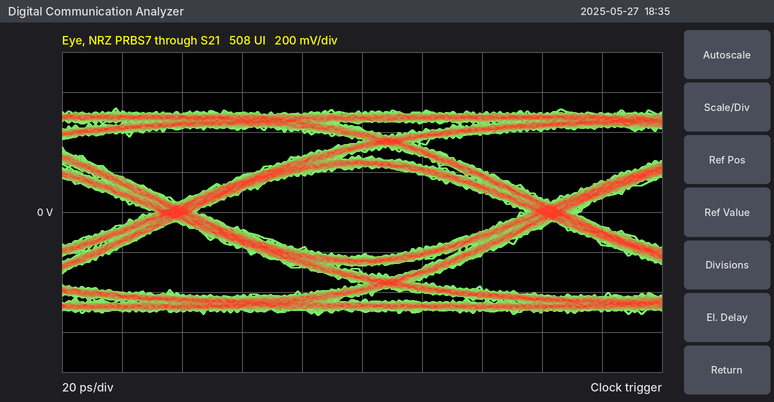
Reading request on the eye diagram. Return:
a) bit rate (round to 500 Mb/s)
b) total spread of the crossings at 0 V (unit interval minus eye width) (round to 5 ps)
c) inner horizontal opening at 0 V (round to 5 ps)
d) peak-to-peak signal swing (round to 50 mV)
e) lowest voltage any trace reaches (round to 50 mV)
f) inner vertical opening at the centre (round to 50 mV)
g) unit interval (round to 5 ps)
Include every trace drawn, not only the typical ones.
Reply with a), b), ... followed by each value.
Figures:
a) 8.0 Gb/s
b) 15 ps
c) 110 ps
d) 1.05 V
e) -500 mV
f) 450 mV
g) 125 ps
